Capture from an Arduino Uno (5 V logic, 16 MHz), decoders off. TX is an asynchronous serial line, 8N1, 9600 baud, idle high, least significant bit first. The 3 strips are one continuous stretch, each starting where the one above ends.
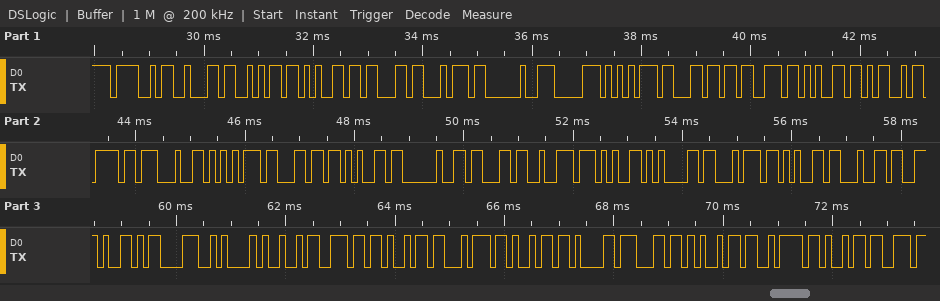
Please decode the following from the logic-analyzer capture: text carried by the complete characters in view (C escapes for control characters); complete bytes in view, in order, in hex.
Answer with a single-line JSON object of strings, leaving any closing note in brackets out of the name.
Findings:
{"text carried by the complete characters in view": "\"Object pulseModule created.\\r\\nInitializi\"", "complete bytes in view, in order, in hex": "4F 62 6A 65 63 74 20 70 75 6C 73 65 4D 6F 64 75 6C 65 20 63 72 65 61 74 65 64 2E 0D 0A 49 6E 69 74 69 61 6C 69 7A 69"}
